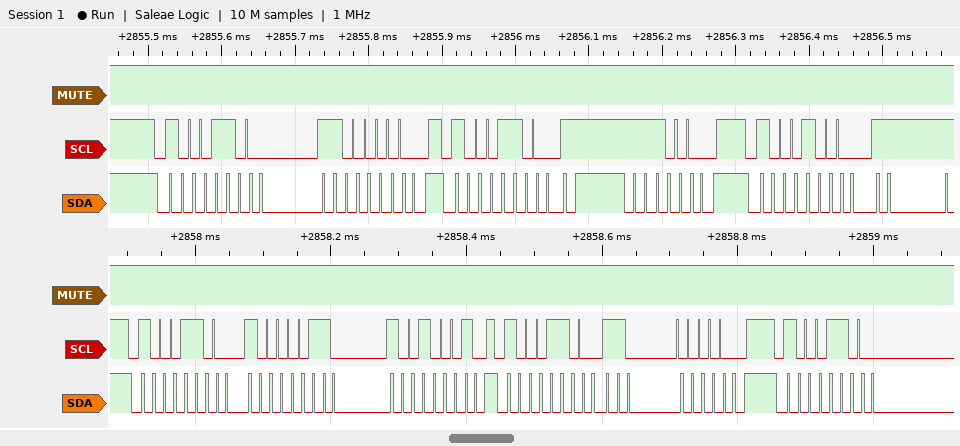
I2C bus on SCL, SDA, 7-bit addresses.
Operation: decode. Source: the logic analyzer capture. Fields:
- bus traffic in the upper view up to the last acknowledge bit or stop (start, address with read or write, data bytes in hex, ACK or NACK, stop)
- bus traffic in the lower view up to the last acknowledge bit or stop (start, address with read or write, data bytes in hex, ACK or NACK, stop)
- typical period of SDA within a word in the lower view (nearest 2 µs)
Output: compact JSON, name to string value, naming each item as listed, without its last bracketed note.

{"bus traffic in the upper view up to the last acknowledge bit or stop": "start, address 46 write ACK, C0 ACK, stop, start, address 46 write ACK, F8 ACK, stop, start, address 44 write ACK", "bus traffic in the lower view up to the last acknowledge bit or stop": "start, address 46 write ACK, 83 ACK, 91 ACK, stop, start, address 46 write ACK, C0 ACK, stop, start, address 46 write ACK", "typical period of SDA within a word in the lower view": "16 µs"}
